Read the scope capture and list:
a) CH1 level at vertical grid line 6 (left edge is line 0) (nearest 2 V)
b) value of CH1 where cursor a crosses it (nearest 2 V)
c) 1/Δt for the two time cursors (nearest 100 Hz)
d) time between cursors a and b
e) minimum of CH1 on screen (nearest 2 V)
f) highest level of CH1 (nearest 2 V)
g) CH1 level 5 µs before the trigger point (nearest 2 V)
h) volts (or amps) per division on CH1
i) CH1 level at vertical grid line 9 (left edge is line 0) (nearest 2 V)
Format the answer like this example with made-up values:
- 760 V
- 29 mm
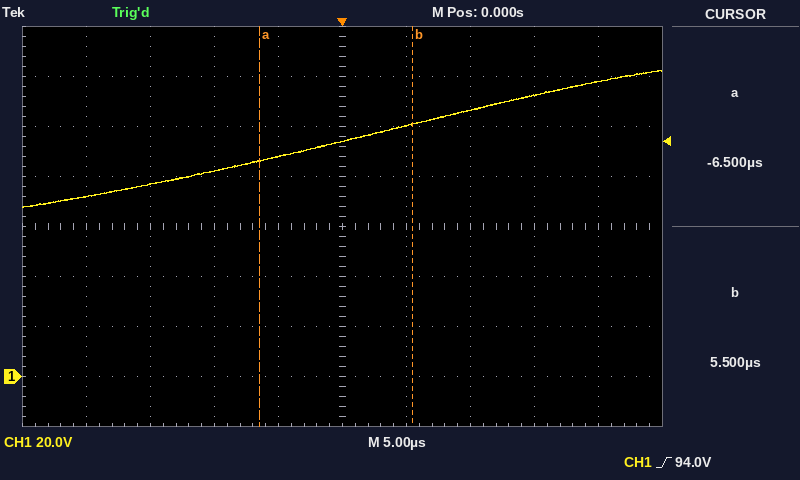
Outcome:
- 100 V
- 86 V
- 83.3 kHz
- 12.0 µs
- 68 V
- 122 V
- 88 V
- 20 V
- 118 V
